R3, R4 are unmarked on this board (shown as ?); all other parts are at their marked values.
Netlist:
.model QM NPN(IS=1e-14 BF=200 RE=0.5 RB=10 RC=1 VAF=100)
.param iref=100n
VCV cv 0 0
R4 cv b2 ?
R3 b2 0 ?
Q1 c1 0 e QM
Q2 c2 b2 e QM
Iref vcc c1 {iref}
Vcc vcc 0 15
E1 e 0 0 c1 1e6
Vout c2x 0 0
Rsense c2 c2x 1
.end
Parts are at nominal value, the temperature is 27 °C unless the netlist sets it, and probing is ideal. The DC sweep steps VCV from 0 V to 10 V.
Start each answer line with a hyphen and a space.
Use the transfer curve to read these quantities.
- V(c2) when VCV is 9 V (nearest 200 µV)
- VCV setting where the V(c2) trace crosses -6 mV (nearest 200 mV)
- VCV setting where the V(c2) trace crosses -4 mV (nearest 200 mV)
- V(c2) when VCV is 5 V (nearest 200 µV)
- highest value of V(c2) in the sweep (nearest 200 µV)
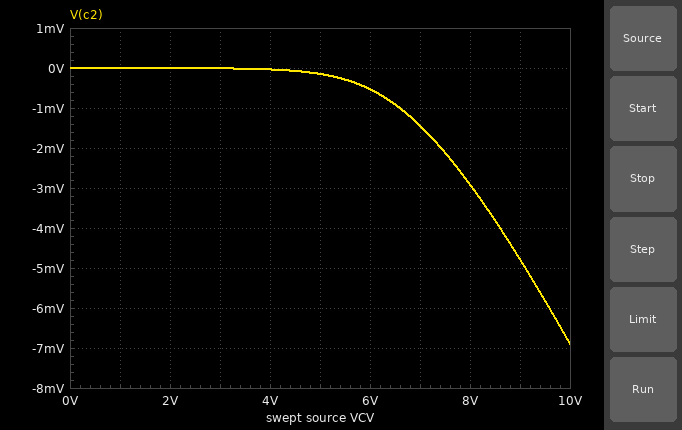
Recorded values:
- -4.8 mV
- 9.6 V
- 8.6 V
- -200 µV
- 0 V
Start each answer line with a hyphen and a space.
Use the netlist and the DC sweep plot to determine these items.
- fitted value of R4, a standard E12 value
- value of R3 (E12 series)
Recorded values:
- 68 kΩ
- 2.7 kΩ
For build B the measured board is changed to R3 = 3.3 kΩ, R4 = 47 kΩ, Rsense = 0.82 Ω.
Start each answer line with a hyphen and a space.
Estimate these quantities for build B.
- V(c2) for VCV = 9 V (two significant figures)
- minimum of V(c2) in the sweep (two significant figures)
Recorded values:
- -14 mV
- -17 mV
